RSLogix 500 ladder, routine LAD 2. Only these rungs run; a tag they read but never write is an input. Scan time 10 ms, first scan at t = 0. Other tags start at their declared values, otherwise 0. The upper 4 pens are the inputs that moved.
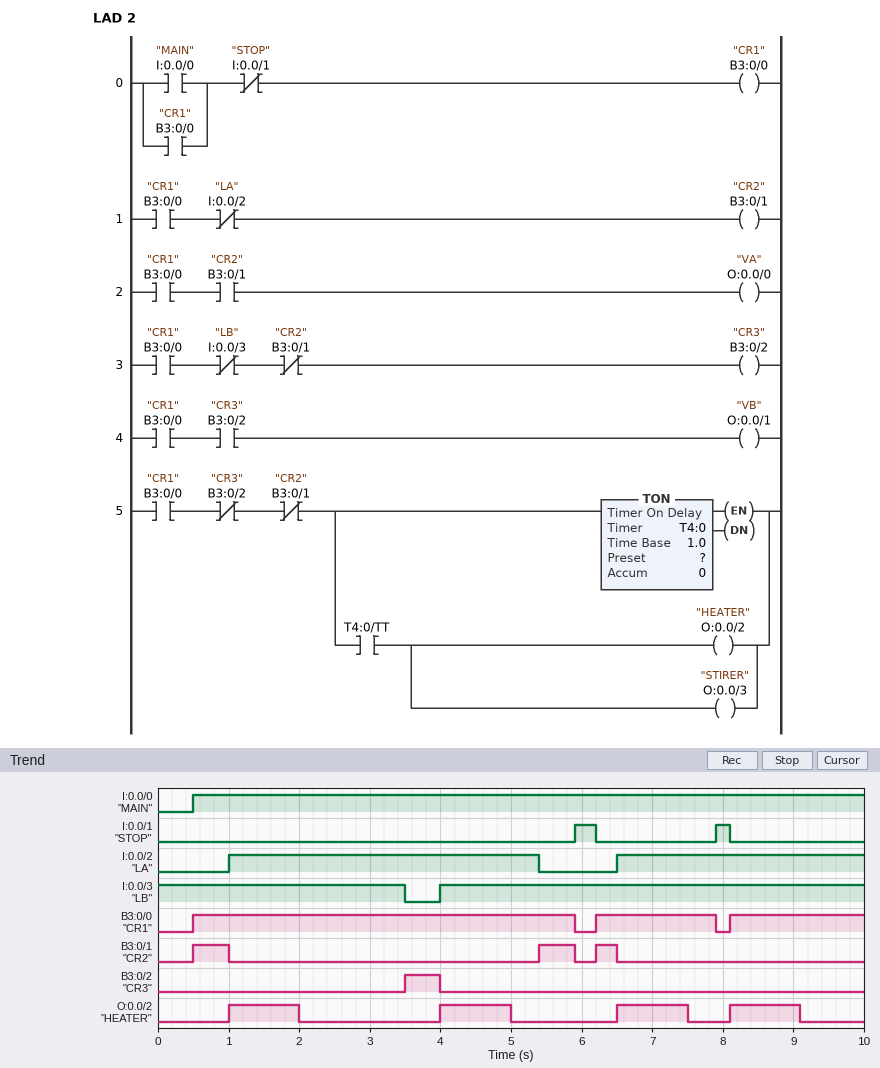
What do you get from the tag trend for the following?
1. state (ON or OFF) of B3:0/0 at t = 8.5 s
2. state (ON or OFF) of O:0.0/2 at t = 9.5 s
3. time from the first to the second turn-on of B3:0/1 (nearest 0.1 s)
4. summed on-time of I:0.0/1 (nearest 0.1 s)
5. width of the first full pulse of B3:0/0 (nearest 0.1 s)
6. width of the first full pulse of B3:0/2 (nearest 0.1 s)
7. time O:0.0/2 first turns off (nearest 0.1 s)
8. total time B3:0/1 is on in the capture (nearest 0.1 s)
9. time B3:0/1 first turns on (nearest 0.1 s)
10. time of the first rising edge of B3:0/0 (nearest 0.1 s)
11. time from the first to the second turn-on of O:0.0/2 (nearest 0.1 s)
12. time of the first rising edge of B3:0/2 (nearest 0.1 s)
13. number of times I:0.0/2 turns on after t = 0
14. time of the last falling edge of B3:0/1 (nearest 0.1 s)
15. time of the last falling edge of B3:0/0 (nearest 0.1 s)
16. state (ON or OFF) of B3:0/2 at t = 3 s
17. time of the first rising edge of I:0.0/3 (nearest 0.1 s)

ON
OFF
4.9 s
0.5 s
5.4 s
0.5 s
2.0 s
1.3 s
0.5 s
0.5 s
3.0 s
3.5 s
2
6.5 s
7.9 s
OFF
4.0 s
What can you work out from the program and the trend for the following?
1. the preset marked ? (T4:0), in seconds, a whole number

1 s
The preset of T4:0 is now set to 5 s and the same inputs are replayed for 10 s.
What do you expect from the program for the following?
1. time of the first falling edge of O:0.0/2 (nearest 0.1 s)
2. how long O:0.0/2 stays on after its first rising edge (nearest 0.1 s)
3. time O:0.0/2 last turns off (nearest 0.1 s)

3.5 s
2.5 s
7.9 s
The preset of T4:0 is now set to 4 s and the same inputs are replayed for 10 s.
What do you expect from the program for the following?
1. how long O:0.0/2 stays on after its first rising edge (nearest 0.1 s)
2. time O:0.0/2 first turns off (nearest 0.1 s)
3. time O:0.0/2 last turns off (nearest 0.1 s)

2.5 s
3.5 s
7.9 s
